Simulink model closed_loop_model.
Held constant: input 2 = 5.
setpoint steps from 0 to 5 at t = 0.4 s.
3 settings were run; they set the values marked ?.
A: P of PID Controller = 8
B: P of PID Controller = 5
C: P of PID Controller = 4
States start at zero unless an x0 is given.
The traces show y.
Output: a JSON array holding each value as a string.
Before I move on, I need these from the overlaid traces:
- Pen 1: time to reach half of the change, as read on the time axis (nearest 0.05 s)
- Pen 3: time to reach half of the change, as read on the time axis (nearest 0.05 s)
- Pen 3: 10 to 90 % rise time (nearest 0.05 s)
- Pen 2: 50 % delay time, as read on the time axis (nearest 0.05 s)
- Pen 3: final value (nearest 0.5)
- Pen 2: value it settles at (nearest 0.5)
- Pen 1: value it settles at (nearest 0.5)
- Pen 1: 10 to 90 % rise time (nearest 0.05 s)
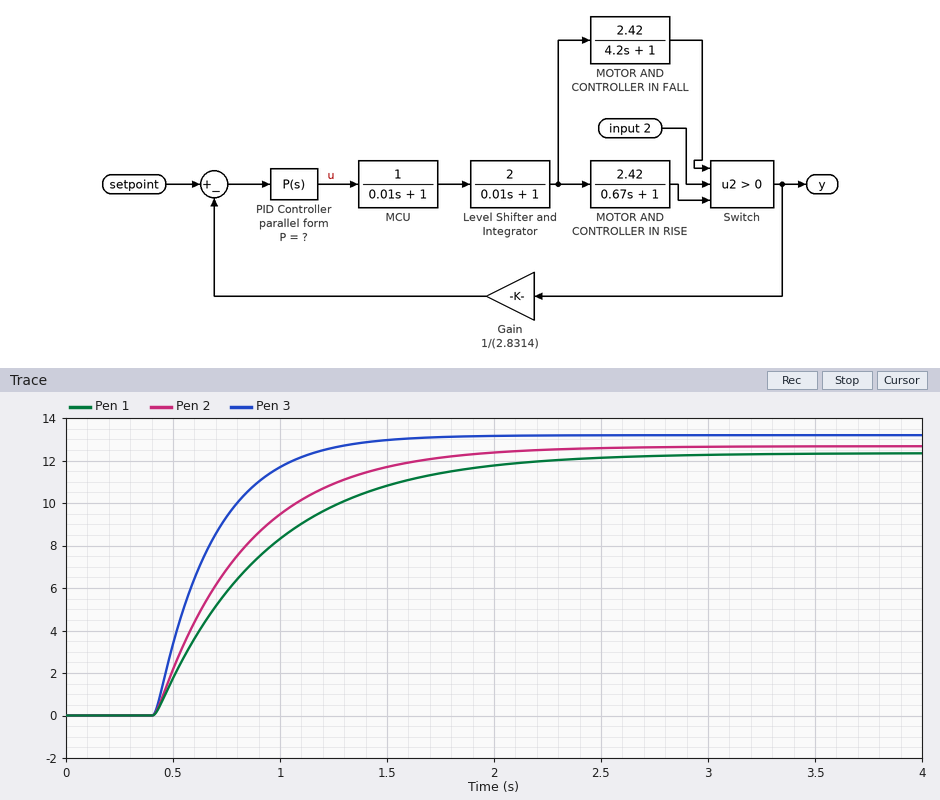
["0.80 s", "0.60 s", "0.60 s", "0.70 s", "13.0", "12.5", "12.5", "1.15 s"]
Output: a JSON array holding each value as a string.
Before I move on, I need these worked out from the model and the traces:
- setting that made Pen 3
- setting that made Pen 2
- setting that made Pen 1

["A", "B", "C"]
